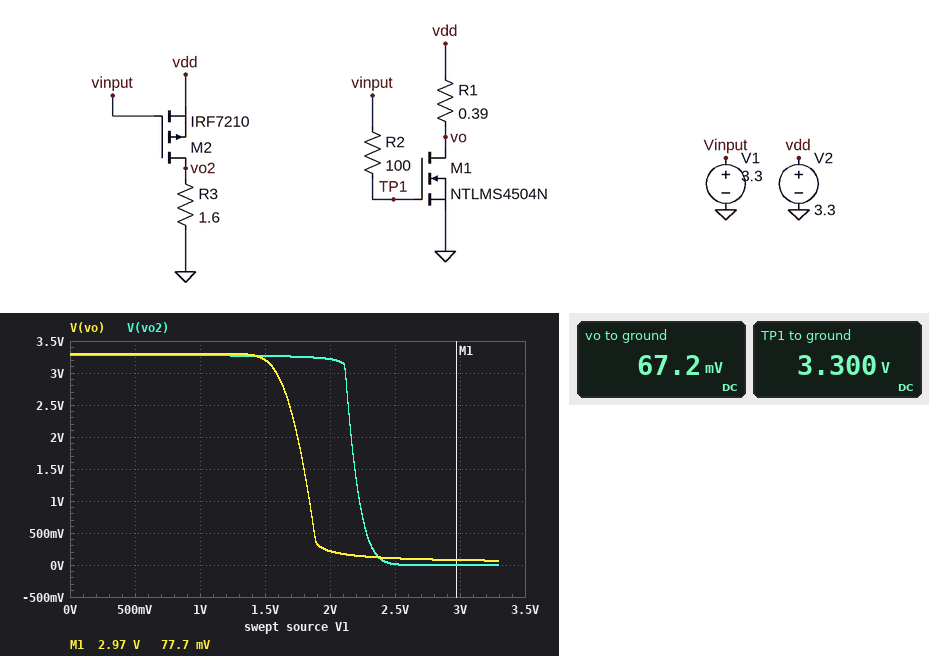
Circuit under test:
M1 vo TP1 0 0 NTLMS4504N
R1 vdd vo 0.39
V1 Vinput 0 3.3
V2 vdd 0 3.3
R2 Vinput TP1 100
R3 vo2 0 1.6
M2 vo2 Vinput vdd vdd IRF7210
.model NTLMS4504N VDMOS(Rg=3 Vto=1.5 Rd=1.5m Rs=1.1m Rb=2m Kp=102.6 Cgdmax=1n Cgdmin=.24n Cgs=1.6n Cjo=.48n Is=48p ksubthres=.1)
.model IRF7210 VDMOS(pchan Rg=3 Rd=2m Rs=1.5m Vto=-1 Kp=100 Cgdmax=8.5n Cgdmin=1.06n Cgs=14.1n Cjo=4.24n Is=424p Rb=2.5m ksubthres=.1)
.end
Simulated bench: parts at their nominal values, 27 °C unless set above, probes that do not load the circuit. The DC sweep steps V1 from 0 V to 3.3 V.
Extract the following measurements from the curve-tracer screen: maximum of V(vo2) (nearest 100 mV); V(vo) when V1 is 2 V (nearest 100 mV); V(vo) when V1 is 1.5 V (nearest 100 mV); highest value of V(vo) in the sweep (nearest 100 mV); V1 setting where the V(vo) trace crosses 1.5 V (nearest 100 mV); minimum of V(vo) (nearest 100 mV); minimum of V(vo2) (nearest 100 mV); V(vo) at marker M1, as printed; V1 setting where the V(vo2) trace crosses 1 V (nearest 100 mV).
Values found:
3.3 V
200 mV
3.2 V
3.3 V
1.8 V
100 mV
0 V
77.7 mV
2.2 V
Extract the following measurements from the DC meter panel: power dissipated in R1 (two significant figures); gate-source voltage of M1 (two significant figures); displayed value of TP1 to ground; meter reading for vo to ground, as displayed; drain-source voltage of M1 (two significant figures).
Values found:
27 W
3.3 V
3.300 V
67.2 mV
67 mV
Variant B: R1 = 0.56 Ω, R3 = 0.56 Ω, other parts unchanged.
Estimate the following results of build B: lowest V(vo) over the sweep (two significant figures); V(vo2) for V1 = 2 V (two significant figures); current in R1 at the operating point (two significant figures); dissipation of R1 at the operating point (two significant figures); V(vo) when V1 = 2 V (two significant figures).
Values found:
47 mV
2.5 V
5.8 A
19 W
140 mV
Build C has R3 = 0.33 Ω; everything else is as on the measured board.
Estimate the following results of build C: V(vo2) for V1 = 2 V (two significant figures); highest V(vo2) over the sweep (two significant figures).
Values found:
1.5 V
3.2 V
